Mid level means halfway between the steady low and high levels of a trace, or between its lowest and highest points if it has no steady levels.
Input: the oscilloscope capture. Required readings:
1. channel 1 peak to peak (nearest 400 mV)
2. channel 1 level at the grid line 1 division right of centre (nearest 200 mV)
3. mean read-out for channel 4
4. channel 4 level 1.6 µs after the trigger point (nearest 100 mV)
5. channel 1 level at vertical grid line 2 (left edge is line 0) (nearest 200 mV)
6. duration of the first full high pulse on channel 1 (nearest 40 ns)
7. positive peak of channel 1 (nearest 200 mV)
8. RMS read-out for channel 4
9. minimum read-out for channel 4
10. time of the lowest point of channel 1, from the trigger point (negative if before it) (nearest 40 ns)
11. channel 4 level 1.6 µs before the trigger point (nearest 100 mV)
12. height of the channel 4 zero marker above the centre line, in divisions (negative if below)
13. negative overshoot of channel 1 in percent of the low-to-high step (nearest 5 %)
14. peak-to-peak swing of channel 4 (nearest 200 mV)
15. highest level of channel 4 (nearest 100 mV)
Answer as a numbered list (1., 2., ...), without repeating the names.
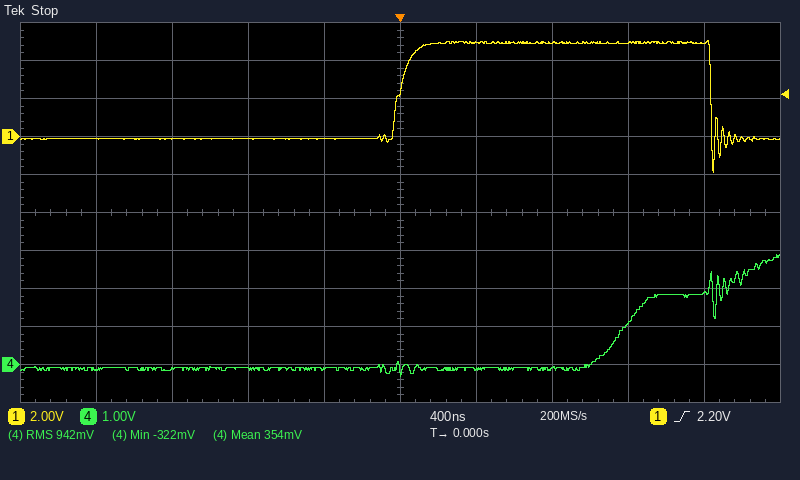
1. 6.8 V
2. 5.0 V
3. 354 mV
4. 1.9 V
5. -200 mV
6. 1.64 µs
7. 5.0 V
8. 942 mV
9. -322 mV
10. +1.64 µs
11. -100 mV
12. -4.0 div
13. 35 %
14. 3.2 V
15. 2.9 V
